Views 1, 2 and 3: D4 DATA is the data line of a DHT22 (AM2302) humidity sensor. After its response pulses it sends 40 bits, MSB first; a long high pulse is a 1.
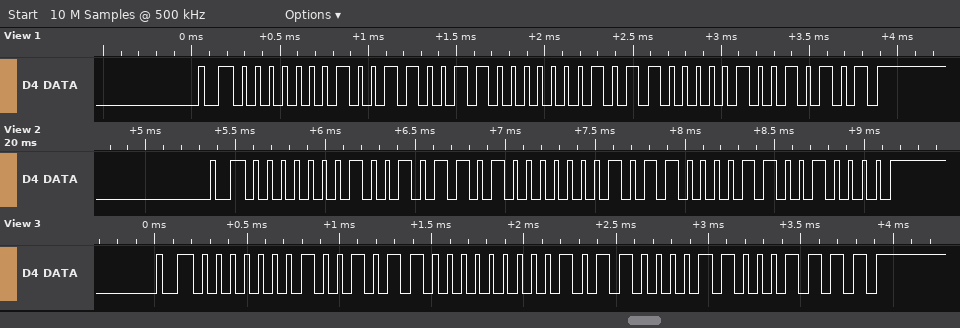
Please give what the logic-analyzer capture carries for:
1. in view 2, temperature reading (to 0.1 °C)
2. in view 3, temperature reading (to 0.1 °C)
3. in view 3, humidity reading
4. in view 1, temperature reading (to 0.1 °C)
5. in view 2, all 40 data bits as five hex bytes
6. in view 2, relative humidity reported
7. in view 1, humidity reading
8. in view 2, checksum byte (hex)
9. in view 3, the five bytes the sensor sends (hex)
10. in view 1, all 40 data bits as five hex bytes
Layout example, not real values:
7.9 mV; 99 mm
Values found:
35.3 °C; 35.3 °C; 30.0 %; 35.2 °C; 01 2D 01 61 90; 30.1 %; 30.7 %; 0x90; 01 2C 01 61 8F; 01 33 01 60 95
